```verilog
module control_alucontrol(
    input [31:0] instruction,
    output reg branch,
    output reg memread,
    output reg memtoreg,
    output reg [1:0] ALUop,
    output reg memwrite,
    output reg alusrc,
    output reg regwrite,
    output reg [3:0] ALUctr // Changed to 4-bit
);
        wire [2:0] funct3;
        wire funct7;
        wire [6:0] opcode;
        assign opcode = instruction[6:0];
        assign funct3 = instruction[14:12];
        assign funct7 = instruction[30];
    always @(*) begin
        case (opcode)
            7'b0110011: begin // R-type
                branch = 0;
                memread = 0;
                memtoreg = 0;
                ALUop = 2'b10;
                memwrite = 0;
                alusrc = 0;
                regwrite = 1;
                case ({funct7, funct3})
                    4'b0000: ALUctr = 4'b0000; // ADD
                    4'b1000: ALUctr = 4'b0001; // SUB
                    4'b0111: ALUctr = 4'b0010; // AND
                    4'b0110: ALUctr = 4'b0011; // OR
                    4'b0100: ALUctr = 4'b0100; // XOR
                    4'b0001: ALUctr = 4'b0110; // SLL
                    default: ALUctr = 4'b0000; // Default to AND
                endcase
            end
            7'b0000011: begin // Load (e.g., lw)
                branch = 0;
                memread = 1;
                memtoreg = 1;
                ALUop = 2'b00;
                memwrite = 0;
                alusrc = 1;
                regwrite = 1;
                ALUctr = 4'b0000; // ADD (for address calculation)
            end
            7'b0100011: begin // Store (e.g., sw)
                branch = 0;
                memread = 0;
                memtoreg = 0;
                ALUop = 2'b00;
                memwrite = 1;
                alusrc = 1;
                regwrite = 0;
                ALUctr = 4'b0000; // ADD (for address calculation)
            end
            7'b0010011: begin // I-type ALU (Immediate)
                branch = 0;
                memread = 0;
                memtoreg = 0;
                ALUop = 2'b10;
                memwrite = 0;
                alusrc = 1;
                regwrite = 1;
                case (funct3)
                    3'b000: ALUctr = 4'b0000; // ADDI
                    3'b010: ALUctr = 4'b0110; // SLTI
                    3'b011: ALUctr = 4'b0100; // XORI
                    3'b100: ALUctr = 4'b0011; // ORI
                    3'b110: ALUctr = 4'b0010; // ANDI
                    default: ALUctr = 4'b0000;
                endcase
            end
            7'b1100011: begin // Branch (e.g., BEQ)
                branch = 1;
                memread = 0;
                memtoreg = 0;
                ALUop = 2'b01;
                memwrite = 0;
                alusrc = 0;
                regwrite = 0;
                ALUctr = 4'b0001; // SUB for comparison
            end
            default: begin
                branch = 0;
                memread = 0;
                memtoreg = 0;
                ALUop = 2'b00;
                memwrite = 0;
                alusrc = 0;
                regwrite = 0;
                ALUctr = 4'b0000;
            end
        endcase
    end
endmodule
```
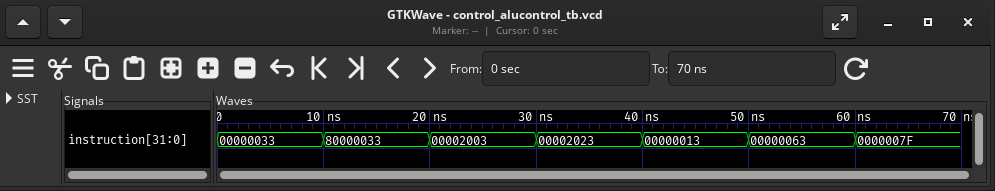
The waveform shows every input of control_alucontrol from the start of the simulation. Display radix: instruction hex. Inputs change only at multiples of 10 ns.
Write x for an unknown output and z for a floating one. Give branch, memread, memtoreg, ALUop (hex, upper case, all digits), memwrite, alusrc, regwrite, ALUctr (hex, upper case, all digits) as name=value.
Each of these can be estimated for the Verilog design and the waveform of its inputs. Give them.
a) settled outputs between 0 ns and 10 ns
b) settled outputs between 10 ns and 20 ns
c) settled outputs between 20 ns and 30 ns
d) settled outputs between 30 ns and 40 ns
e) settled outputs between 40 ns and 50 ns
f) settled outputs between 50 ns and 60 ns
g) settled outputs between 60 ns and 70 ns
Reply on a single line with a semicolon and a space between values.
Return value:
branch=0, memread=0, memtoreg=0, ALUop=2, memwrite=0, alusrc=0, regwrite=1, ALUctr=0; branch=0, memread=0, memtoreg=0, ALUop=2, memwrite=0, alusrc=0, regwrite=1, ALUctr=0; branch=0, memread=1, memtoreg=1, ALUop=0, memwrite=0, alusrc=1, regwrite=1, ALUctr=0; branch=0, memread=0, memtoreg=0, ALUop=0, memwrite=1, alusrc=1, regwrite=0, ALUctr=0; branch=0, memread=0, memtoreg=0, ALUop=2, memwrite=0, alusrc=1, regwrite=1, ALUctr=0; branch=1, memread=0, memtoreg=0, ALUop=1, memwrite=0, alusrc=0, regwrite=0, ALUctr=1; branch=0, memread=0, memtoreg=0, ALUop=0, memwrite=0, alusrc=0, regwrite=0, ALUctr=0
